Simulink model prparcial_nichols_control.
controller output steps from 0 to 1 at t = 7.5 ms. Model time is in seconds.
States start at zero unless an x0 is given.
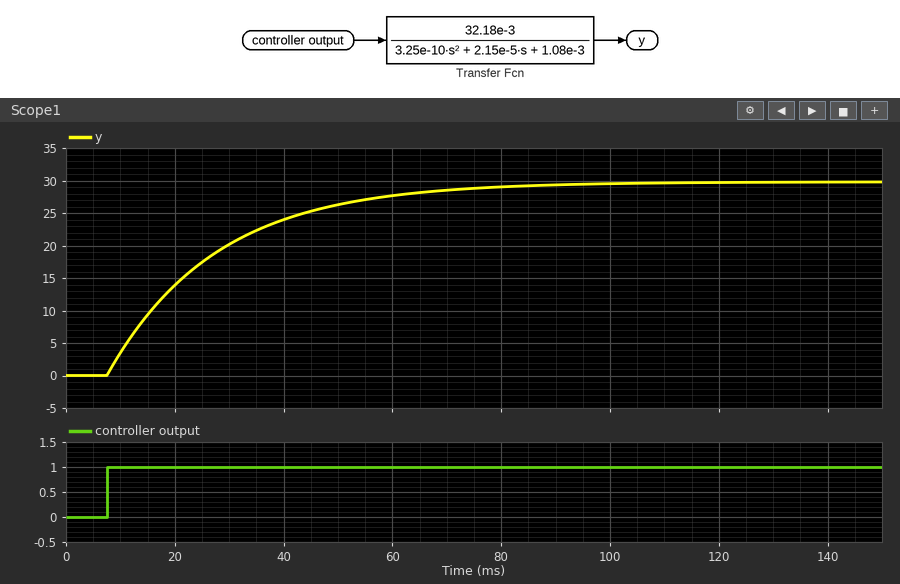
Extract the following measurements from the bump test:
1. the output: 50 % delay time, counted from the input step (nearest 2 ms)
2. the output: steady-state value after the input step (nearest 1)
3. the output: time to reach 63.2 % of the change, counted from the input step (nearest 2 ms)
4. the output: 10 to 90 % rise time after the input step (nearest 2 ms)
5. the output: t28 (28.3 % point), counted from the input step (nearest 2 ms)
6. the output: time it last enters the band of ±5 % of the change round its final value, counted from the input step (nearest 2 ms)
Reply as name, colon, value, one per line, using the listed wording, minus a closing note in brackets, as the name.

the output: 50 % delay time, counted from the input step: 14 ms
the output: steady-state value after the input step: 30
the output: time to reach 63.2 % of the change, counted from the input step: 20 ms
the output: 10 to 90 % rise time after the input step: 44 ms
the output: t28 (28.3 % point), counted from the input step: 6 ms
the output: time it last enters the band of ±5 % of the change round its final value, counted from the input step: 60 ms
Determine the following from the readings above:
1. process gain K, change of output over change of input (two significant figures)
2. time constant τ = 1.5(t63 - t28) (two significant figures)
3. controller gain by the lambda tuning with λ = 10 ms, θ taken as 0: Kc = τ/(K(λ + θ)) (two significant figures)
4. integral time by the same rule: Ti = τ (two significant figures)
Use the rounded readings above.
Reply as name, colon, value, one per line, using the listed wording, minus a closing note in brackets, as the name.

process gain K, change of output over change of input: 30
time constant τ = 1.5(t63 - t28): 21 ms
controller gain by the lambda tuning with λ = 10 ms, θ taken as 0: Kc = τ/(K(λ + θ)): 0.070
integral time by the same rule: Ti = τ: 21 ms
